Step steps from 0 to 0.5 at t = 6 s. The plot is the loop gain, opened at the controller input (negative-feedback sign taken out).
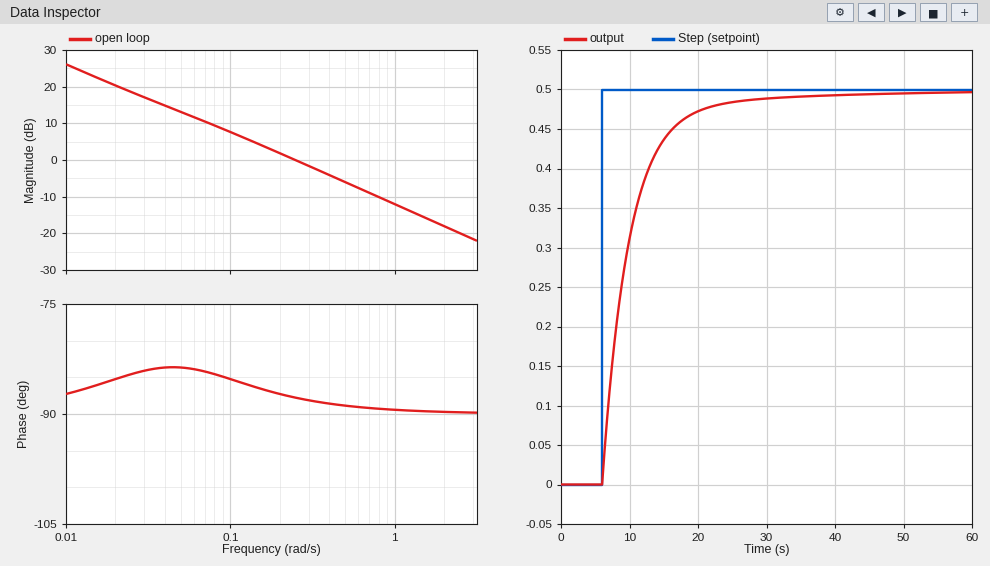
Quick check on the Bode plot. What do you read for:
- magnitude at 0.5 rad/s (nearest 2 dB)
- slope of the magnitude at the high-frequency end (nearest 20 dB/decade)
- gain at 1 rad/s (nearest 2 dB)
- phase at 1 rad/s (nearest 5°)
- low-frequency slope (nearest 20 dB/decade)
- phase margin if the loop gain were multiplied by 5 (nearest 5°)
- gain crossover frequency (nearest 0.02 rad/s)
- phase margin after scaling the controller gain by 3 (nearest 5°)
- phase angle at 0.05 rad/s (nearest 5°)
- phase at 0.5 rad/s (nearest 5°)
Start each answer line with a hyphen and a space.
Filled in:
- -6 dB
- -20 dB/decade
- -12 dB
- -90°
- -20 dB/decade
- 90°
- 0.24 rad/s
- 90°
- -85°
- -90°
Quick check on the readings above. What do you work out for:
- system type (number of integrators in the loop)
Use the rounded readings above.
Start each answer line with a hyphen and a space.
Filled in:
- 1
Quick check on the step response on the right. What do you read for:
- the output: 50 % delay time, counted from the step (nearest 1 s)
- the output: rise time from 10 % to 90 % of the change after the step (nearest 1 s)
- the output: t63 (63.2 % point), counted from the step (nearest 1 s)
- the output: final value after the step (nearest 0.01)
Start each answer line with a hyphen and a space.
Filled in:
- 3 s
- 10 s
- 4 s
- 0.50
